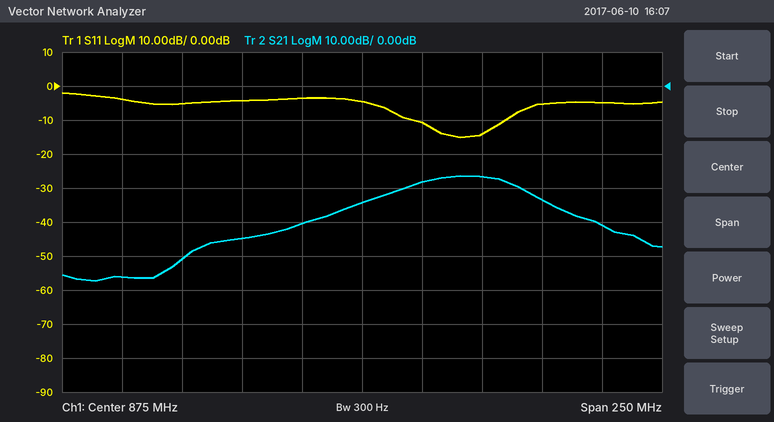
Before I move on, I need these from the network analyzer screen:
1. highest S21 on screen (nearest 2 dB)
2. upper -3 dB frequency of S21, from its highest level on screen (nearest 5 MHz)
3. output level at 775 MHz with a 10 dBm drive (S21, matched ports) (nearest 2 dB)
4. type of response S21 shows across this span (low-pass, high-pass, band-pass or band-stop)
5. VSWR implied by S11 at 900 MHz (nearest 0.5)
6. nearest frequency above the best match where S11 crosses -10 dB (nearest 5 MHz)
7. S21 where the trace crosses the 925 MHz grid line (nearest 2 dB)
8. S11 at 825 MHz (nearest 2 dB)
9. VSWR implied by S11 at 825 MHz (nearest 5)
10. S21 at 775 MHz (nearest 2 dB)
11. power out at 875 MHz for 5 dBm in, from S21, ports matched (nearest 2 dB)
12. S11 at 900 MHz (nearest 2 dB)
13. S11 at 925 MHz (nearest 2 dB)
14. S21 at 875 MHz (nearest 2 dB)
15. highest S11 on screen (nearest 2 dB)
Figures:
-26 dB
940 MHz
-46 dBm
band-pass
2.0
935 MHz
-26 dB
-4 dB
5
-56 dB
-30 dBm
-10 dB
-14 dB
-34 dB
-2 dB
